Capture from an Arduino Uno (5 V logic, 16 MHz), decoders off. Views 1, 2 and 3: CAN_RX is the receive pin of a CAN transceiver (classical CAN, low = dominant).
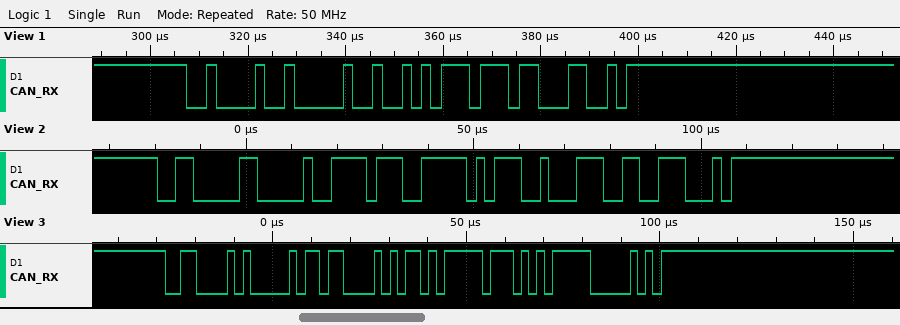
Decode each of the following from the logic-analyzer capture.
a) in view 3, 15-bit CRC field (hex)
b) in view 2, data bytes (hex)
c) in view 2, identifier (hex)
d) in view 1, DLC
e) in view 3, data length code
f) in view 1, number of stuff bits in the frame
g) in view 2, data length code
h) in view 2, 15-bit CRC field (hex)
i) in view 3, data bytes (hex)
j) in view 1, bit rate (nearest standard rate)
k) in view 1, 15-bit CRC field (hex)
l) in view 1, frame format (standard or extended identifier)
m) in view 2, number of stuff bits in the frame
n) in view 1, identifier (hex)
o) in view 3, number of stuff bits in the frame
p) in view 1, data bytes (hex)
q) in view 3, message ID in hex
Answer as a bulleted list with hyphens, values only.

- 0x2BE0
- DC FD C8
- 0x304
- 1
- 3
- 1
- 3
- 0x7338
- 61 5A FF
- 500 kbit/s
- 0x5D8C
- standard
- 3
- 0x212
- 4
- 2B
- 0x30A
